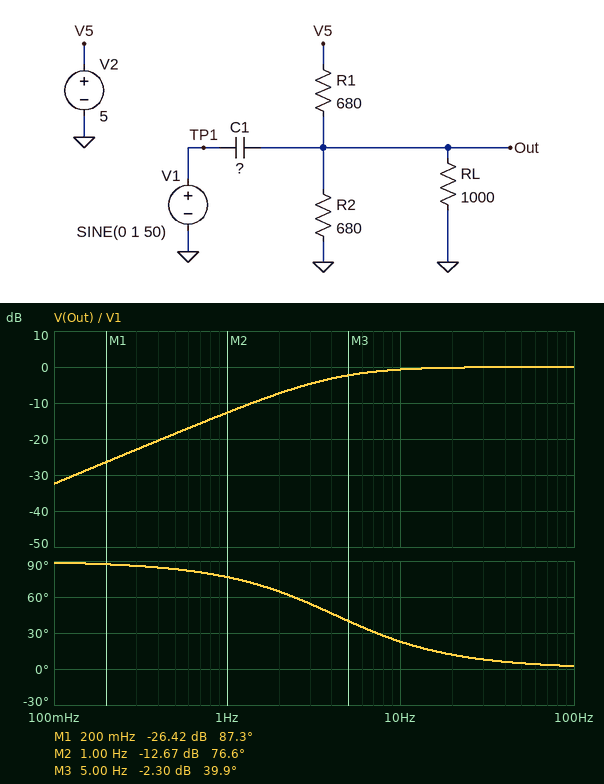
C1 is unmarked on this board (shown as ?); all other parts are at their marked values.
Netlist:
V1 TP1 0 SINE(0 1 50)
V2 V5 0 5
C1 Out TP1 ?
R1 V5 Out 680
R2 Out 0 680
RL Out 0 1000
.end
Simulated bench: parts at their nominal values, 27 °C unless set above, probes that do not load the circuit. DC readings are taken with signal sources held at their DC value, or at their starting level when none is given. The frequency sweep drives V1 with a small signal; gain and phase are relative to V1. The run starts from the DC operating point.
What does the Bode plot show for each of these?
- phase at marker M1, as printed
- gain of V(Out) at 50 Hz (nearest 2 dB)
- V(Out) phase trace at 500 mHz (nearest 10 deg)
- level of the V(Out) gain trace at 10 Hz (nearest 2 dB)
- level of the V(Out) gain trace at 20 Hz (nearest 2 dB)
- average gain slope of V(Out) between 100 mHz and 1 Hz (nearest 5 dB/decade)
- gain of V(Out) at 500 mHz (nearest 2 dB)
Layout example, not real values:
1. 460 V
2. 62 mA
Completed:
1. 87.3 deg
2. 0 dB
3. 80 deg
4. 0 dB
5. 0 dB
6. 20 dB/decade
7. -18 dB
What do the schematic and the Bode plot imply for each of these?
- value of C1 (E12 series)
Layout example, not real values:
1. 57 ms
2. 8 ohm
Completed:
1. 150 µF
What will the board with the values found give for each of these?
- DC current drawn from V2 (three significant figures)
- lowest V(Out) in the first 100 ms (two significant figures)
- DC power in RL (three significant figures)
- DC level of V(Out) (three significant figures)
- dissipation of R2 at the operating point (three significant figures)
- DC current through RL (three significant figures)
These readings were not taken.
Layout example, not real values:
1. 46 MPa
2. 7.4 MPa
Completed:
1. 4.61 mA
2. 810 mV
3. 3.48 mW
4. 1.87 V
5. 5.12 mW
6. 1.87 mA
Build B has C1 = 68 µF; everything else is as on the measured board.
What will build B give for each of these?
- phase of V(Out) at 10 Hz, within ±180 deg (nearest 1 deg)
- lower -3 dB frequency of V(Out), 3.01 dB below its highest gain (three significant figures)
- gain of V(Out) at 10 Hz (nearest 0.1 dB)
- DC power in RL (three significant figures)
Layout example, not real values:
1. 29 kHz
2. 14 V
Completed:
1. 43 deg
2. 9.22 Hz
3. -2.7 dB
4. 3.48 mW
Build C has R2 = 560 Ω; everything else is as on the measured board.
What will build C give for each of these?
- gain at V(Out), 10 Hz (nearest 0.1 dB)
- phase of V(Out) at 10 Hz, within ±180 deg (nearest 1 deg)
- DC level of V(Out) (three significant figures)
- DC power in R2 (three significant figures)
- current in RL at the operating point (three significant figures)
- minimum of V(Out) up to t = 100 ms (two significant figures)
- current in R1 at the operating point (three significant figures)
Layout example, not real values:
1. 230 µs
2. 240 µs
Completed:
1. -0.8 dB
2. 24 deg
3. 1.73 V
4. 5.33 mW
5. 1.73 mA
6. 670 mV
7. 4.81 mA
